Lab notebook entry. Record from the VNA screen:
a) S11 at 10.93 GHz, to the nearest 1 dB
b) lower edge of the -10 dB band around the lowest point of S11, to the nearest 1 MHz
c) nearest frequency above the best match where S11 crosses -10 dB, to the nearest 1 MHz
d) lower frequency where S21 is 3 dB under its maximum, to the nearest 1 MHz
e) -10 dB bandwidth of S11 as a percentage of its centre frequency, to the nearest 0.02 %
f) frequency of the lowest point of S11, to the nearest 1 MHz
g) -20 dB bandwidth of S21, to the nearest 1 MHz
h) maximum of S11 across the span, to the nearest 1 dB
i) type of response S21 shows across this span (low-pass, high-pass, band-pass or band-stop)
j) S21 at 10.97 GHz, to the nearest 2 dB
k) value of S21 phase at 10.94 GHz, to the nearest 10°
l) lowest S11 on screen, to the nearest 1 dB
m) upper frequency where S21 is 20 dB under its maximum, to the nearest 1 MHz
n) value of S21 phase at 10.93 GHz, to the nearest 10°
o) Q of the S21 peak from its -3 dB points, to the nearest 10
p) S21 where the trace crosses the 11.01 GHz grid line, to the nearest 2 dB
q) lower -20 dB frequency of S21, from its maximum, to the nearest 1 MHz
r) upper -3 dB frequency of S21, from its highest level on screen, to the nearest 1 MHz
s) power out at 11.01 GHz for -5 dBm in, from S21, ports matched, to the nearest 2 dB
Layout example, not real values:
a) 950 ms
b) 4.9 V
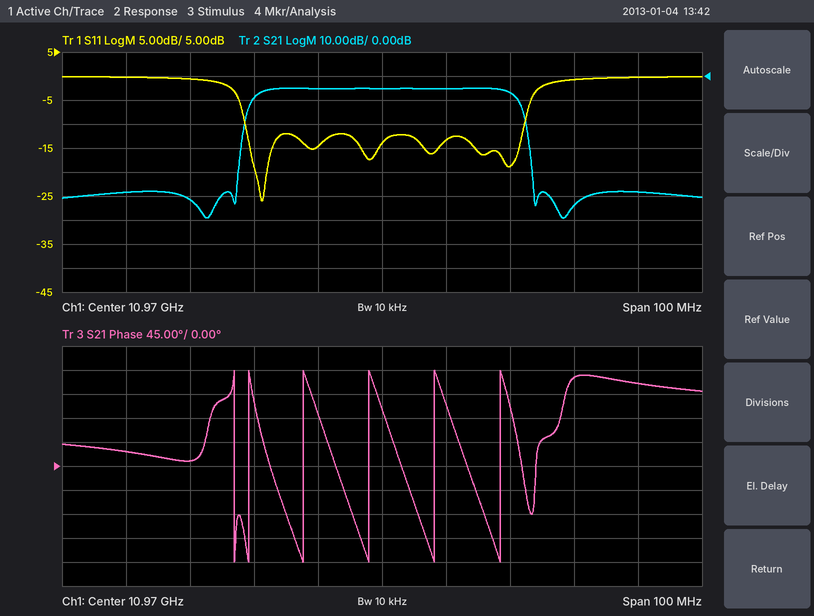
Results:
a) 0 dB
b) 10.949 GHz
c) 10.992 GHz
d) 10.950 GHz
e) 0.40 %
f) 10.951 GHz
g) 45 MHz
h) 0 dB
i) band-pass
j) -6 dB
k) 10°
l) -26 dB
m) 10.993 GHz
n) 30°
o) 270
p) -48 dB
q) 10.948 GHz
r) 10.991 GHz
s) -54 dBm
